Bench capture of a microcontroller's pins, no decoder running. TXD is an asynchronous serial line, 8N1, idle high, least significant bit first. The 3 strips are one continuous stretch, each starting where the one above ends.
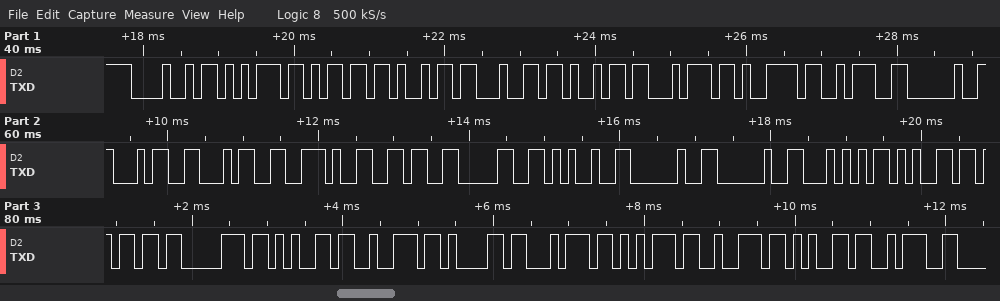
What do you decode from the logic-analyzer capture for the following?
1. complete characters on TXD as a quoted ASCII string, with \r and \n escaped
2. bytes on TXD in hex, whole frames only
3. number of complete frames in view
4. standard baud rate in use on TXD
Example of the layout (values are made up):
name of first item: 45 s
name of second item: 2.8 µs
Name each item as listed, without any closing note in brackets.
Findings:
complete characters on TXD as a quoted ASCII string, with \r and \n escaped: "Humidity: 44.60%  Temperature:"
bytes on TXD in hex, whole frames only: 48 75 6D 69 64 69 74 79 3A 20 34 34 2E 36 30 25 20 20 54 65 6D 70 65 72 61 74 75 72 65 3A
number of complete frames in view: 30
standard baud rate in use on TXD: 9600 baud
